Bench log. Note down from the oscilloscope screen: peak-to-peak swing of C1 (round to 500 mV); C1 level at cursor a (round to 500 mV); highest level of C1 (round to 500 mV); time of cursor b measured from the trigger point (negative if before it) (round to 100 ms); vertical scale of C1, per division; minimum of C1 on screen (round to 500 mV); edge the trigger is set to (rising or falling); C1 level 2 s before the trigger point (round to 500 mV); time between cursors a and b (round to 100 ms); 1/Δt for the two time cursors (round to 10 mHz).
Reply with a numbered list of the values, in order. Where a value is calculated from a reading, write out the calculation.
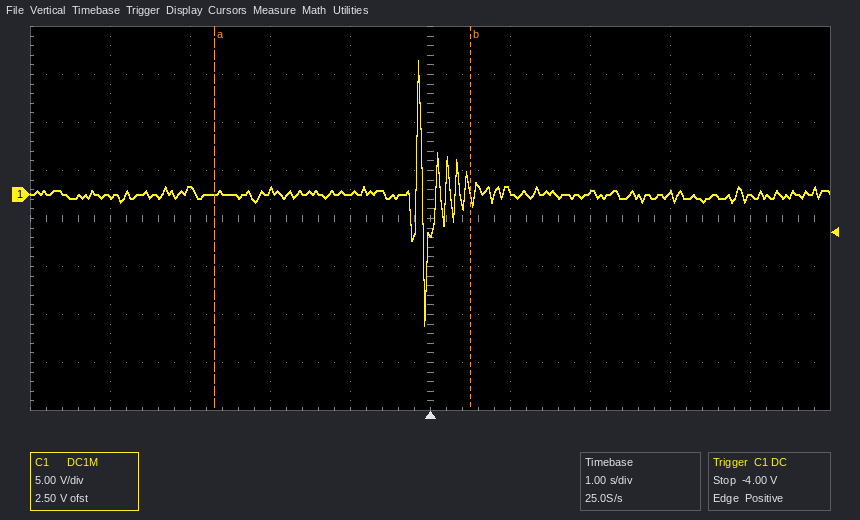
1. 14.0 V − (-13.5 V) = 27.5 V
2. 0.0 V
3. 14.0 V
4. +500 ms
5. 5 V
6. -13.5 V
7. rising
8. 500 mV
9. 3.2 s
10. 1 / 3.2 s ≈ 310 mHz
